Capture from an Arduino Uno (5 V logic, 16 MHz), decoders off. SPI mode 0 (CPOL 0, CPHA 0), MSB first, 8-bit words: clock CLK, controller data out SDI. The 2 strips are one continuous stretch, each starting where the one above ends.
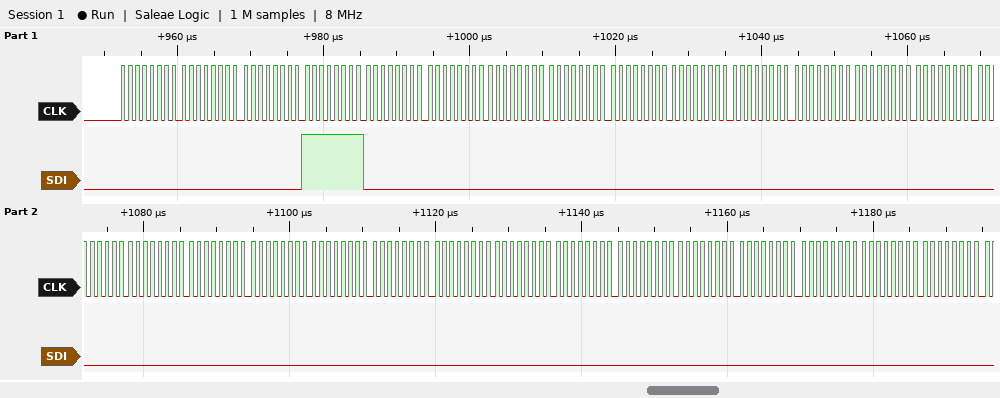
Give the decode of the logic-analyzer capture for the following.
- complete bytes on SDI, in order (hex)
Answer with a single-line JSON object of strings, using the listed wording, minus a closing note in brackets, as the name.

{"complete bytes on SDI, in order": "0x00 0x00 0x00 0xFF 0x00 0x00 0x00 0x00 0x00 0x00 0x00 0x00 0x00 0x00 0x00 0x00 0x00 0x00 0x00 0x00 0x00 0x00 0x00 0x00 0x00 0x00 0x00 0x00 0x00"}
